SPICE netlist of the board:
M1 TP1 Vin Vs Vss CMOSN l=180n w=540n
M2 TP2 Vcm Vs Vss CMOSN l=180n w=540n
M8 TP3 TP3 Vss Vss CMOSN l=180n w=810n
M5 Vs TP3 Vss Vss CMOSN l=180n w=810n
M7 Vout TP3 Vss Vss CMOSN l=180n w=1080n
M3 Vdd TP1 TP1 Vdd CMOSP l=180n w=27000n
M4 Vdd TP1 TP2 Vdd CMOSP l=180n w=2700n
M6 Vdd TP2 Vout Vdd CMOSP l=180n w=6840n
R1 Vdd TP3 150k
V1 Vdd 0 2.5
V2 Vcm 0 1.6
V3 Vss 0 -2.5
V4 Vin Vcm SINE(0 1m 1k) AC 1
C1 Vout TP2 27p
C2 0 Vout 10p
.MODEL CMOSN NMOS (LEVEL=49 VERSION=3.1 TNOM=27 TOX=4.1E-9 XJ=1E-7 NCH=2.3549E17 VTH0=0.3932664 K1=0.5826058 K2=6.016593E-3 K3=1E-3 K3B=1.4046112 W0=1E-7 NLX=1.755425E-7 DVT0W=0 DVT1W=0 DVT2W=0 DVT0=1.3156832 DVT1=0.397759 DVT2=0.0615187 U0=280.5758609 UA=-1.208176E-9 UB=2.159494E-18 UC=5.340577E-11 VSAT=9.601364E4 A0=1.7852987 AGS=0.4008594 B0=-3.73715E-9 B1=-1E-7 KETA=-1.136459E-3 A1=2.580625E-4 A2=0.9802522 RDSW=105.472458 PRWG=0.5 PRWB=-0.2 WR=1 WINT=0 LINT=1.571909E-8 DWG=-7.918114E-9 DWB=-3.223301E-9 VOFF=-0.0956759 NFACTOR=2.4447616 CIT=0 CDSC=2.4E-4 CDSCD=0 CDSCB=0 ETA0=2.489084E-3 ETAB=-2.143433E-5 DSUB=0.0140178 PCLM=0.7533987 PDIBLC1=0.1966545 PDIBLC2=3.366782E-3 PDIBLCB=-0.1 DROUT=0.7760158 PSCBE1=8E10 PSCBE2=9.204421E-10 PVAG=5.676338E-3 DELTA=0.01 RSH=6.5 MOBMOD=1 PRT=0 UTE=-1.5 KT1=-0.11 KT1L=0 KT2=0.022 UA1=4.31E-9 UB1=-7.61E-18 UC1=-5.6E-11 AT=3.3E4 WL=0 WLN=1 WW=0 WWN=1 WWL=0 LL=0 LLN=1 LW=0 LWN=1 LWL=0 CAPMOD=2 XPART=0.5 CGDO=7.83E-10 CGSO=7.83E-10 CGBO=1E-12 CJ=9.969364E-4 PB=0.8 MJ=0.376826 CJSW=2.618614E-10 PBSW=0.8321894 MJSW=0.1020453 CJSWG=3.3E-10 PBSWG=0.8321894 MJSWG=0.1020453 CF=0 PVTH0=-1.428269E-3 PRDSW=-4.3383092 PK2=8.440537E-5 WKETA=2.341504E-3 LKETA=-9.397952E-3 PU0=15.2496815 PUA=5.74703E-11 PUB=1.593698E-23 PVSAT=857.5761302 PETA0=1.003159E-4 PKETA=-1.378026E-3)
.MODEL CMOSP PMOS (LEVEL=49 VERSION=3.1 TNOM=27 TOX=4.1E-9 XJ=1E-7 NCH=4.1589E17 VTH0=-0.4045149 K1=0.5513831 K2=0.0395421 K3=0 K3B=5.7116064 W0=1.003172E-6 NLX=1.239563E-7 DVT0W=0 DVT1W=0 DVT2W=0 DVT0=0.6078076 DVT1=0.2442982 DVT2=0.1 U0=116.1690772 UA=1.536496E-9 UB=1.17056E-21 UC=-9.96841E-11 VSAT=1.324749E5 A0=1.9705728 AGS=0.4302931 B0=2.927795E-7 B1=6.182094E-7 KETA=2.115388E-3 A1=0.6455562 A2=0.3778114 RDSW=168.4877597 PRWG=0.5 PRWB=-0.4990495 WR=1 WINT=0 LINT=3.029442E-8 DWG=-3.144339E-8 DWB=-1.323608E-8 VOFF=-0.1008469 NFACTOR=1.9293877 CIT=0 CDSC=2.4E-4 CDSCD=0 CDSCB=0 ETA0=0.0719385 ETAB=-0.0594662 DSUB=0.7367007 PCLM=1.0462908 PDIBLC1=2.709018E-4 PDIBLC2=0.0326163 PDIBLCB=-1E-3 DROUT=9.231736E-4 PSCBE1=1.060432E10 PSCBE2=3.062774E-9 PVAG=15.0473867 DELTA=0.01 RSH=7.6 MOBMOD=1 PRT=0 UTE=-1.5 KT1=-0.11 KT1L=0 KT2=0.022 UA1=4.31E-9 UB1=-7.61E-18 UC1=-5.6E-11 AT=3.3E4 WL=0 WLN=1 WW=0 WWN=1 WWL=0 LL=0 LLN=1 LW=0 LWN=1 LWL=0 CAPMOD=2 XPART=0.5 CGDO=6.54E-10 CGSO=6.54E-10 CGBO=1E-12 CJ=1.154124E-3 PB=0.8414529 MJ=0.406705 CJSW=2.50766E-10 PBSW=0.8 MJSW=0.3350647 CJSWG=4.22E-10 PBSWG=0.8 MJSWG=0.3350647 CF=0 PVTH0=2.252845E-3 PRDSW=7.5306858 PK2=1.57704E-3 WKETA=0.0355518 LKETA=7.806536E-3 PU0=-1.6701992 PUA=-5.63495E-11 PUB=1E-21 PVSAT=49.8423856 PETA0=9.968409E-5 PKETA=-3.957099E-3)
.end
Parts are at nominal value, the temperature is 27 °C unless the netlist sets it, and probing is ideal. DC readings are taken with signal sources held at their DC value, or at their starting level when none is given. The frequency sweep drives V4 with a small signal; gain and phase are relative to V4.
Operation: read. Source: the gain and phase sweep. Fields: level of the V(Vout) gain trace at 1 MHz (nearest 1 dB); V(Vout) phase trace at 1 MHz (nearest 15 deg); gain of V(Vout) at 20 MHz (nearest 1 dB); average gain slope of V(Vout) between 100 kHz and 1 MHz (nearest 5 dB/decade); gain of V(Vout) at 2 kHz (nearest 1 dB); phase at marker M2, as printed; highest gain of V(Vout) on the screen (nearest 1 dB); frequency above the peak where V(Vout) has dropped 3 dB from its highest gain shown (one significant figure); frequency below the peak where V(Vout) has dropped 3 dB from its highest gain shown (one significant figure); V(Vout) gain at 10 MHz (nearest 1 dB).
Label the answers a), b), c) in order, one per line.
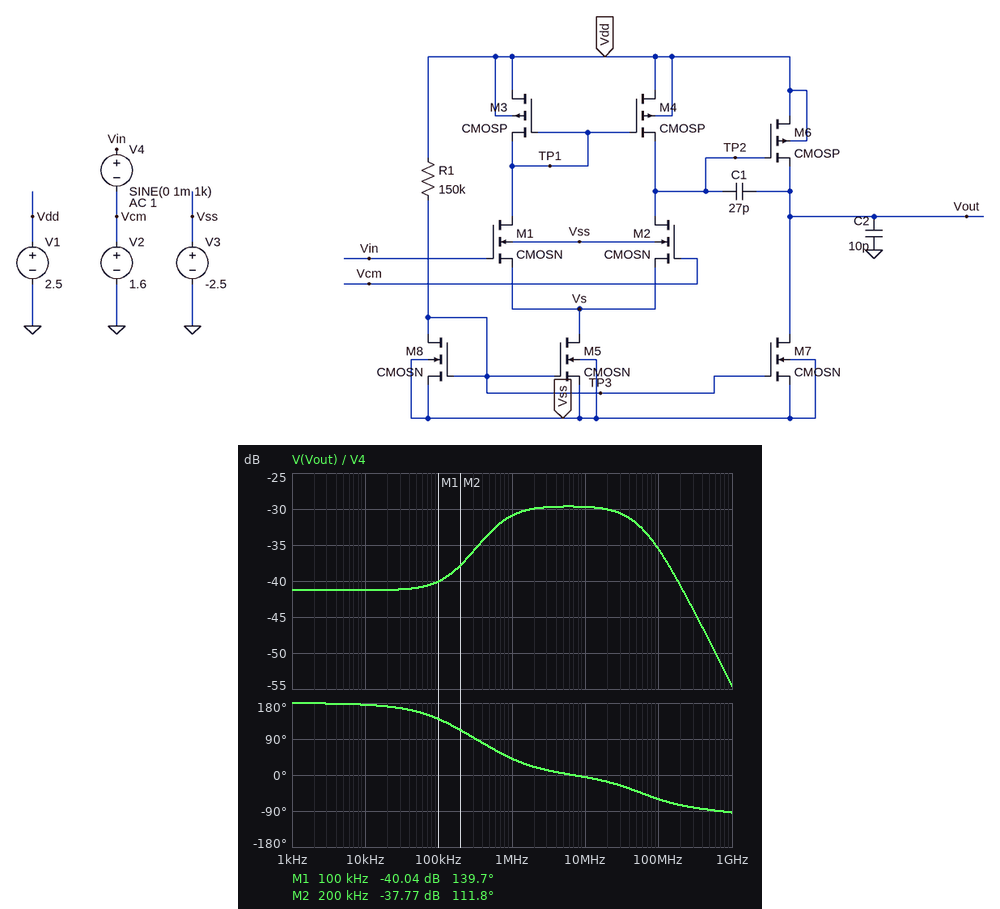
a) -31 dB
b) 45 deg
c) -30 dB
d) 10 dB/decade
e) -41 dB
f) 111.8 deg
g) -30 dB
h) 60 MHz
i) 600 kHz
j) -30 dB
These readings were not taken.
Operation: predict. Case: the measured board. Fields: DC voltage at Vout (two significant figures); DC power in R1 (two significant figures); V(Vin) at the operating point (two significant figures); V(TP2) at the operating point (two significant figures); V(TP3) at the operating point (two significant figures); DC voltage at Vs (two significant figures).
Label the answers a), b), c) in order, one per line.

a) 2.5 V
b) 120 µW
c) 1.6 V
d) 390 mV
e) -1.8 V
f) 340 mV
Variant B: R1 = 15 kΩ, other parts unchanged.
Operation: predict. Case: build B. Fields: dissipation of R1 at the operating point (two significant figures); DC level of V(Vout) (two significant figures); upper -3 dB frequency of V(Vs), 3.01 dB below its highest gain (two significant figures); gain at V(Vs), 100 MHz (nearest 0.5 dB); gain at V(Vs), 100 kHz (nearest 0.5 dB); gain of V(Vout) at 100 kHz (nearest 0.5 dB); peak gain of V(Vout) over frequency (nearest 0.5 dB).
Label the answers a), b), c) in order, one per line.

a) 940 µW
b) 2.4 V
c) 1.9 MHz
d) -10.0 dB
e) -2.5 dB
f) -35.0 dB
g) -25.5 dB
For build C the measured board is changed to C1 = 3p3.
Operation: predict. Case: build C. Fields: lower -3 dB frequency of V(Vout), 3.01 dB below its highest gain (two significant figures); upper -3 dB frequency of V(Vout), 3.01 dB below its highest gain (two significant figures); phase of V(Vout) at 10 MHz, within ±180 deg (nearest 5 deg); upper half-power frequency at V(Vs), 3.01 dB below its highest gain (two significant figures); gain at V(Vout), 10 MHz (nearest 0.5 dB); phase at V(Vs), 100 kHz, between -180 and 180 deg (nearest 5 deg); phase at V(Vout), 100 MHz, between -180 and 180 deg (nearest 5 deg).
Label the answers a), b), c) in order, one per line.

a) 4.1 MHz
b) 67 MHz
c) 25 deg
d) 9.8 MHz
e) -30.5 dB
f) 0 deg
g) -55 deg
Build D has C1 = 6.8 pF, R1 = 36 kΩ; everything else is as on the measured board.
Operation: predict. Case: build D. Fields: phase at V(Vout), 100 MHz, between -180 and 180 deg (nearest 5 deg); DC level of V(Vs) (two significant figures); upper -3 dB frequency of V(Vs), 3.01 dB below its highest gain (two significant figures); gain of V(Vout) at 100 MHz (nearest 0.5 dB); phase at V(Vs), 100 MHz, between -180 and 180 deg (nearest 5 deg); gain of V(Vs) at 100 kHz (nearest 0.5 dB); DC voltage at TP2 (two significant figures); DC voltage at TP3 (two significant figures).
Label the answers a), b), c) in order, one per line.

a) -55 deg
b) 100 mV
c) 6.5 MHz
d) -32.0 dB
e) -5 deg
f) -2.0 dB
g) 160 mV
h) -1.6 V
